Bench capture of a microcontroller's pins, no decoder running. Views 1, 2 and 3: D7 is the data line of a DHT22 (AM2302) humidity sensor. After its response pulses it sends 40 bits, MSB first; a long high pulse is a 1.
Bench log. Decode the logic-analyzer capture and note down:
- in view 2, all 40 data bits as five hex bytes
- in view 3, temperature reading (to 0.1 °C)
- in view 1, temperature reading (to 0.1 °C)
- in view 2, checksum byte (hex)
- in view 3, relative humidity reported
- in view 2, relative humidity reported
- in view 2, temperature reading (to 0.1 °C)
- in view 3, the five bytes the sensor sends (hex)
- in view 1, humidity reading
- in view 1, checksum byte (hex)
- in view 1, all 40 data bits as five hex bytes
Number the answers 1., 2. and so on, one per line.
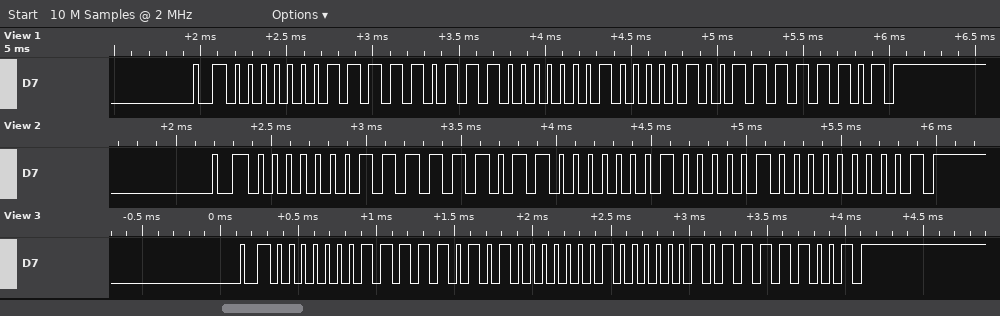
1. 01 FB 01 04 01
2. 25.8 °C
3. 26.0 °C
4. 0x01
5. 50.1 %
6. 50.7 %
7. 26.0 °C
8. 01 F5 01 02 F9
9. 50.3 %
10. 0xFD
11. 01 F7 01 04 FD
